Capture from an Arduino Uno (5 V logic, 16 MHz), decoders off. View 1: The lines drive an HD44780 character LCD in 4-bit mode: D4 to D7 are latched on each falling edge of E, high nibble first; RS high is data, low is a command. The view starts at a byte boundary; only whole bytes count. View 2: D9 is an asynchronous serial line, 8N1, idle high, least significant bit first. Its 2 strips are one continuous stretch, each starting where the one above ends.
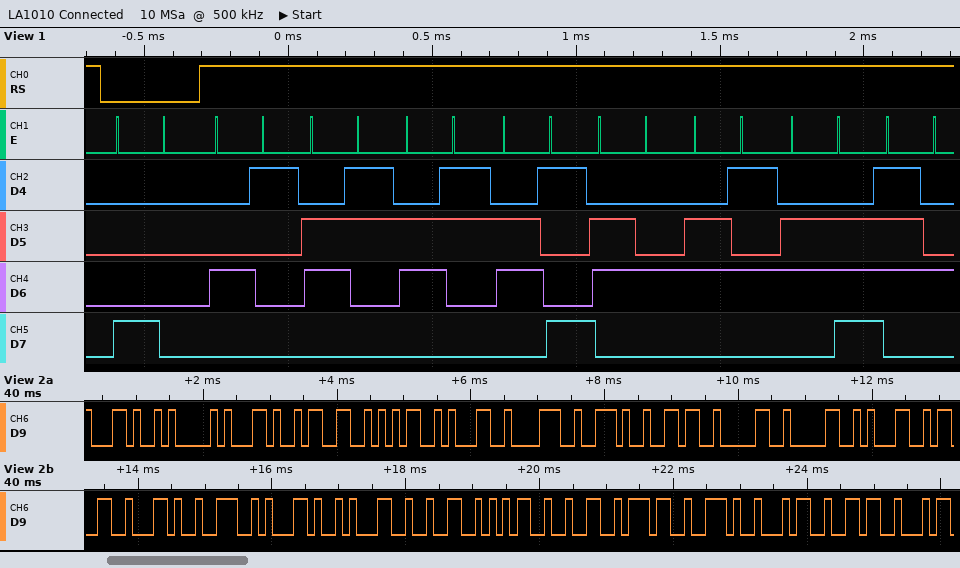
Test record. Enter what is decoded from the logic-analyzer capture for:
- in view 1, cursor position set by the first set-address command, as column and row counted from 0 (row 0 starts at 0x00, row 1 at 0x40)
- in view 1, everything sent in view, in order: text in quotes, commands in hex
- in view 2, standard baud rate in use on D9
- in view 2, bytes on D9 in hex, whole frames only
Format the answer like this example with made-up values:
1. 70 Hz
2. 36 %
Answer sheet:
1. column 0, row 0
2. 0x80 "Accident"
3. 9600 baud
4. 2C 41 2C 33 35 31 38 2E 36 30 30 31 33 2C 4E 2C 31 32 35 32 37 2E 34 36
